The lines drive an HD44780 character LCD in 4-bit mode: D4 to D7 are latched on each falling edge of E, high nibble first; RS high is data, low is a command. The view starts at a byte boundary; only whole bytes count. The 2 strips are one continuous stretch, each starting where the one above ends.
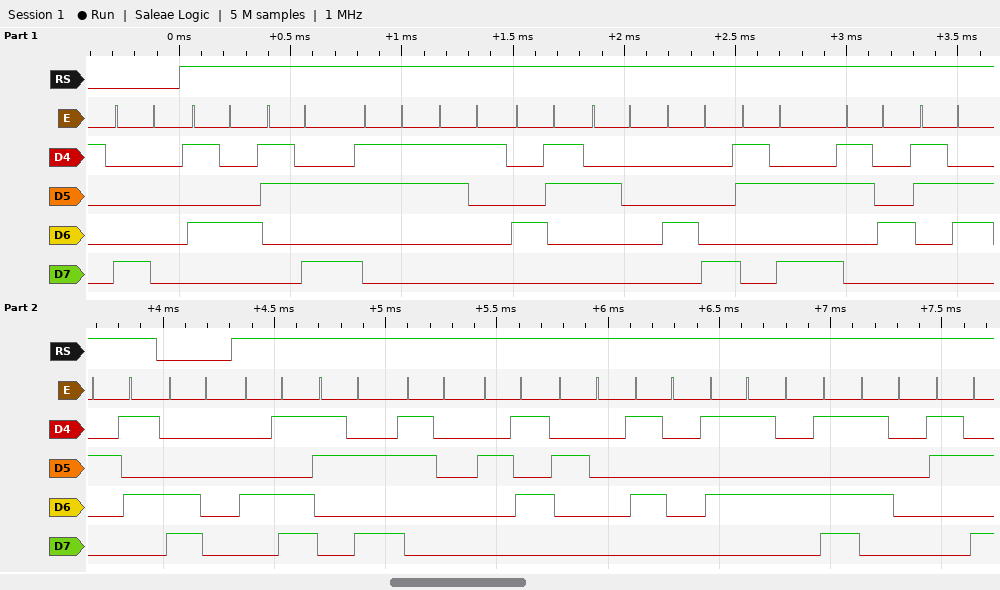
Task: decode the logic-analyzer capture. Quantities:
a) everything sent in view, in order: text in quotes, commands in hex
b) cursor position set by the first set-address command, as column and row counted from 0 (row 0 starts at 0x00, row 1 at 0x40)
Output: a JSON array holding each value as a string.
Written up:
["0x80 \"T:31C H:46%\" 0xC0 \"M:0% PUMP:\"", "column 0, row 0"]
